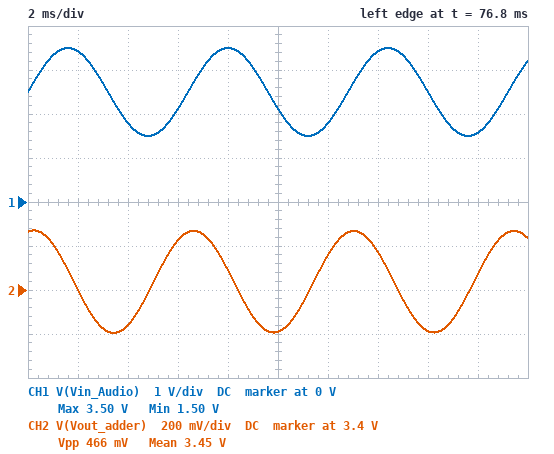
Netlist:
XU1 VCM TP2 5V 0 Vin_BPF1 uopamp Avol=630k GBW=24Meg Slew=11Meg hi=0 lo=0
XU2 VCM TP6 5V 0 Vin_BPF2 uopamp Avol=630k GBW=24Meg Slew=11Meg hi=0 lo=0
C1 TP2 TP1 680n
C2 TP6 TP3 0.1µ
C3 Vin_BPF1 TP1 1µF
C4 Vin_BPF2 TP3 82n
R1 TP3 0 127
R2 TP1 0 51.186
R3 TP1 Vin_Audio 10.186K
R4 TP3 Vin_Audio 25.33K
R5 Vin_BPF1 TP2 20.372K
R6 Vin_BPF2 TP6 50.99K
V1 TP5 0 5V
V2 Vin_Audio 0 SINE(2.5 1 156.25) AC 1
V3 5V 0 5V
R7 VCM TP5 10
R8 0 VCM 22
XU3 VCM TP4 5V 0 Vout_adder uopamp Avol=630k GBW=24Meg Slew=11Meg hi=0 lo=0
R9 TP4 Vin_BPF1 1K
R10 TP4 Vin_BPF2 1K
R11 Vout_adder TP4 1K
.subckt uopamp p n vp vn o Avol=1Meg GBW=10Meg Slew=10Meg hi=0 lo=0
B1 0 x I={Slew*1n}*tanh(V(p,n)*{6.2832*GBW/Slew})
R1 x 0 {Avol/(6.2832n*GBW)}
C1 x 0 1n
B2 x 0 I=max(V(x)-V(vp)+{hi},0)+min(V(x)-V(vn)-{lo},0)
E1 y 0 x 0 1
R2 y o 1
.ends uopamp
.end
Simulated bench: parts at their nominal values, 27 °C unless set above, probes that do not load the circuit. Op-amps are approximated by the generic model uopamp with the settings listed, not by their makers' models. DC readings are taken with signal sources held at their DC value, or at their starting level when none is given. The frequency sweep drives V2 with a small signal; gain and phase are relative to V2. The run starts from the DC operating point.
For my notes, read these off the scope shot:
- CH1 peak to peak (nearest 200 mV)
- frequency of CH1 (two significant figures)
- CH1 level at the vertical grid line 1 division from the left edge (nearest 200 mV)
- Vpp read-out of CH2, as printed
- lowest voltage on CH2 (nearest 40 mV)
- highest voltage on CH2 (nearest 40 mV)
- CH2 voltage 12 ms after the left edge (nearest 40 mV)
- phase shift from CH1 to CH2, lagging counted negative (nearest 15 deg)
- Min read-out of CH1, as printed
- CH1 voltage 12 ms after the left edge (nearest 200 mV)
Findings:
2.0 V
160 Hz
3.4 V
466 mV
3.20 V
3.68 V
3.56 V
75 deg
1.50 V
1.8 V
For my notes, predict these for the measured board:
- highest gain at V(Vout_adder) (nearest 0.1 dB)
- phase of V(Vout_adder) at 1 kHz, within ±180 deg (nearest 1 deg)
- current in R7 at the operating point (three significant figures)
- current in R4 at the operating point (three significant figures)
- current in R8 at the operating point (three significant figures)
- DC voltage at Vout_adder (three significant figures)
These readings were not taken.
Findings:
0.9 dB
-83 deg
156 mA
98.2 µA
156 mA
3.44 V
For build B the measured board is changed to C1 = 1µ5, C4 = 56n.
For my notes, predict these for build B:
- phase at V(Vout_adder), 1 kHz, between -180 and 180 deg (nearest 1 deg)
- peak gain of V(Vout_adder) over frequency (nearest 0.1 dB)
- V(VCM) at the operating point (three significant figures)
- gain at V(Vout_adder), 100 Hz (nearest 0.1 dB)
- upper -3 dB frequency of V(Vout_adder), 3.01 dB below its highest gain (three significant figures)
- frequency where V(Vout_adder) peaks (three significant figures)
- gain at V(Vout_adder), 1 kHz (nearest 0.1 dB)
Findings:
-74 deg
2.2 dB
3.44 V
-11.7 dB
883 Hz
838 Hz
-8.5 dB
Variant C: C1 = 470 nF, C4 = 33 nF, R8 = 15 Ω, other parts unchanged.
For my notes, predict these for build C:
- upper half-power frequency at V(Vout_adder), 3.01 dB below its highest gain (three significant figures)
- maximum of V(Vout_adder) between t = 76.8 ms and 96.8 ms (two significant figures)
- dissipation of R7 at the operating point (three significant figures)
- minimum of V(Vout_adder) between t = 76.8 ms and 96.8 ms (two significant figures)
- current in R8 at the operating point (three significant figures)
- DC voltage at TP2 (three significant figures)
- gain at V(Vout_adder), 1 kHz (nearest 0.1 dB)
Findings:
1.16 kHz
3.1 V
400 mW
2.9 V
200 mA
3.00 V
-1.7 dB
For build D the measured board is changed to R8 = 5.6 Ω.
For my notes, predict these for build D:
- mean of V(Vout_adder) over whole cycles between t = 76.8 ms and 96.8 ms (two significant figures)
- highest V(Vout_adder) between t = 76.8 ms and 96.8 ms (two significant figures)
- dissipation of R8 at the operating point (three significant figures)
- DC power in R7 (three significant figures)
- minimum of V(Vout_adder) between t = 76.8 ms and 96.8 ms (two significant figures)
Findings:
1.8 V
2.0 V
575 mW
1.03 W
1.6 V
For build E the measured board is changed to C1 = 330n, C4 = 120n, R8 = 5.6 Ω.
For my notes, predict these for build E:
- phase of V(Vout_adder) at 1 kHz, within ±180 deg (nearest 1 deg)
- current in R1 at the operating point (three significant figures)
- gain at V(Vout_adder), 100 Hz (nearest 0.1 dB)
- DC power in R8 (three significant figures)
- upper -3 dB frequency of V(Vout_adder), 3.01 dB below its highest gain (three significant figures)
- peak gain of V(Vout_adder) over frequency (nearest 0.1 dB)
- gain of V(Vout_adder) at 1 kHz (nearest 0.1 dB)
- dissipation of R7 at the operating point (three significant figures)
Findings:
-86 deg
98.2 µA
-27.8 dB
575 mW
604 Hz
-0.7 dB
-20.5 dB
1.03 W
